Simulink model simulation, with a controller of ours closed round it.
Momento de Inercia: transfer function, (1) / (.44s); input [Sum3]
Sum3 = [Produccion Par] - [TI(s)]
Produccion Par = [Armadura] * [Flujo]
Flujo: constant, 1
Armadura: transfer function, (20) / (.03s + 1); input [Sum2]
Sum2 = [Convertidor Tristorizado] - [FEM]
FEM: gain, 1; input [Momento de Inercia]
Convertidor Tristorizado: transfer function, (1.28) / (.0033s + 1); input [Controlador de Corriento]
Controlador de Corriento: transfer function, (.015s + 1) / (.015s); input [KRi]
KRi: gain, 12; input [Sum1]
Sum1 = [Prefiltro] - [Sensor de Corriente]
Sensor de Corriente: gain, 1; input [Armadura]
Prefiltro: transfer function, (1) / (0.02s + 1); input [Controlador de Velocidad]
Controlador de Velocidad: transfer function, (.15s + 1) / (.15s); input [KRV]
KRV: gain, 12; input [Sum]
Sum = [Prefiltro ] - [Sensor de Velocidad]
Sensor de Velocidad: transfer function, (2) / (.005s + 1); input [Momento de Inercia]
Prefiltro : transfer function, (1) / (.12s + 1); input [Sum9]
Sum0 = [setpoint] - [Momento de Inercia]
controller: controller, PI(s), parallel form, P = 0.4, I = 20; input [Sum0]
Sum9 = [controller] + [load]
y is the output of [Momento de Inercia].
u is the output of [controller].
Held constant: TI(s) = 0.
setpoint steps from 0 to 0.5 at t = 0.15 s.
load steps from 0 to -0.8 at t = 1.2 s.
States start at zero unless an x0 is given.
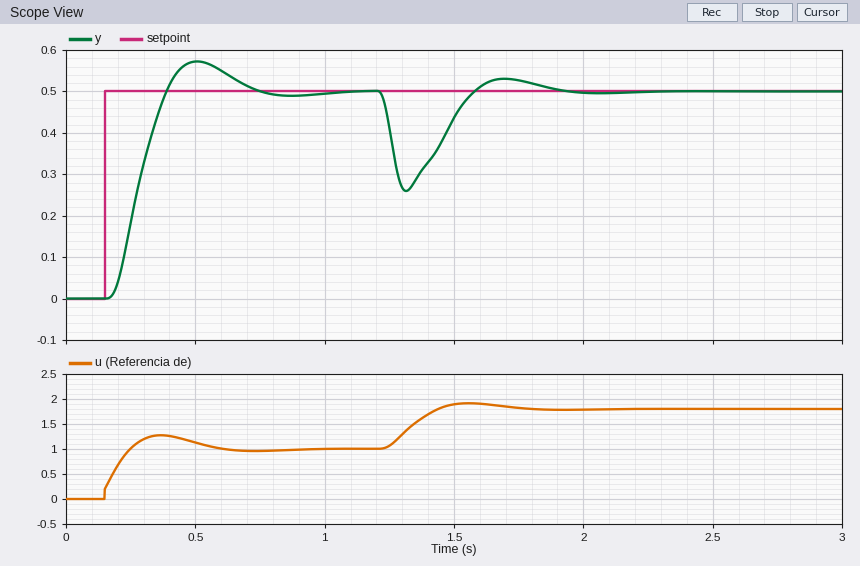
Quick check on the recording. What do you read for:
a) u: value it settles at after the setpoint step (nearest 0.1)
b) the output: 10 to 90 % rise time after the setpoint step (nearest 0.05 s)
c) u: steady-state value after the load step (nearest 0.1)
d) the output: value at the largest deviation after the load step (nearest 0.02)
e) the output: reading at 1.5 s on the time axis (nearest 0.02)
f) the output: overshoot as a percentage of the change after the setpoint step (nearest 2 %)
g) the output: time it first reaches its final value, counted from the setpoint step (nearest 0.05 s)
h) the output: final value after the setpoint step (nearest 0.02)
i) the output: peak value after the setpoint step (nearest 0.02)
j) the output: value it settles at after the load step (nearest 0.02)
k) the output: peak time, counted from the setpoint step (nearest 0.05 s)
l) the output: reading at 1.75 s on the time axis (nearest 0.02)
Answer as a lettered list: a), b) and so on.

a) 1.0
b) 0.15 s
c) 1.8
d) 0.26
e) 0.44
f) 14 %
g) 0.25 s
h) 0.50
i) 0.58
j) 0.50
k) 0.35 s
l) 0.52
